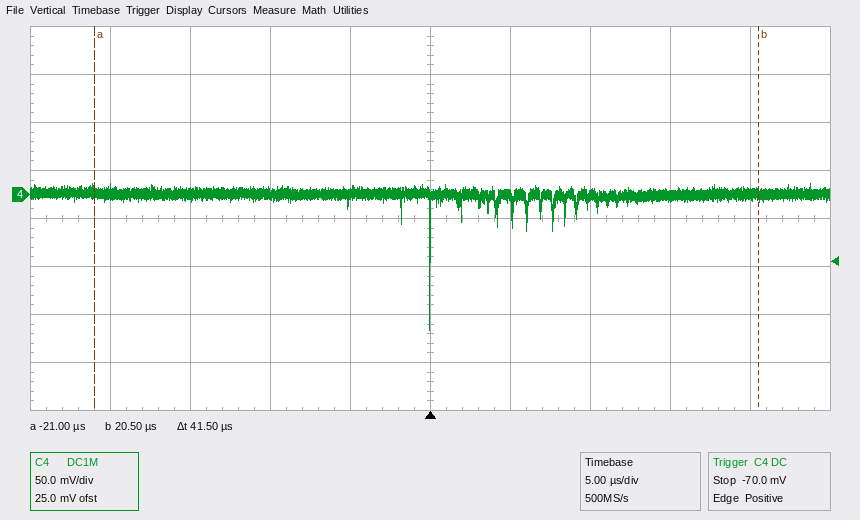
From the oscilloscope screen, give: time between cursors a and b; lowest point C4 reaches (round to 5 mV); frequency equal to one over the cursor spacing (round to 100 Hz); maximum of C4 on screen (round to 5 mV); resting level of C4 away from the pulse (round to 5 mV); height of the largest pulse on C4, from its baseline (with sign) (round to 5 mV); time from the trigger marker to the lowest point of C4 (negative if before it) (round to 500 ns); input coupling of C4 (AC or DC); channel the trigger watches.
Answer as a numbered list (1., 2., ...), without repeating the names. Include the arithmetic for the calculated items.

1. 41.5 µs
2. -140 mV
3. 1 / 41.5 µs ≈ 24.1 kHz
4. 10 mV
5. 0 mV
6. -140 mV − (0 mV) = -140 mV
7. 0.0 µs
8. DC
9. C4
